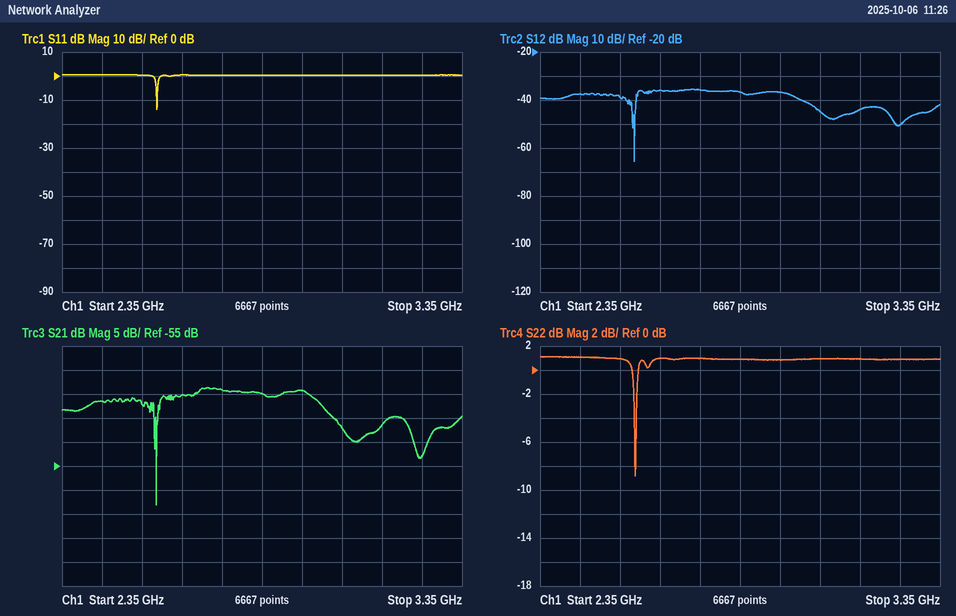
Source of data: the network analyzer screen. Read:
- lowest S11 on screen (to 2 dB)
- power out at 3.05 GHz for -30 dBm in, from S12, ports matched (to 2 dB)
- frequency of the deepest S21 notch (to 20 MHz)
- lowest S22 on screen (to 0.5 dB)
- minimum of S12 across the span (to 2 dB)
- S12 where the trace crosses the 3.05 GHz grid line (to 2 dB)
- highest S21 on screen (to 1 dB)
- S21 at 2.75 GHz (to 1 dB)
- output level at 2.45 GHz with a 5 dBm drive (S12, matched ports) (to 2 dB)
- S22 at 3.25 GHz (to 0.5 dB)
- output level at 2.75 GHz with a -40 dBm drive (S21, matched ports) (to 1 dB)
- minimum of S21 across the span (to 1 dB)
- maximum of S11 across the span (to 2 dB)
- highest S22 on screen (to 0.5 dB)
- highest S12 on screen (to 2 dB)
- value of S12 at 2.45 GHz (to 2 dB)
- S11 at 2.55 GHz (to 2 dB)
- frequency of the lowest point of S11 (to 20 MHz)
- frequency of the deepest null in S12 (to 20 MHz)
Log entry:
-14 dB
-74 dBm
2.58 GHz
-9.0 dB
-66 dB
-44 dB
-39 dB
-39 dB
-32 dBm
1.0 dB
-79 dBm
-63 dB
0 dB
1.0 dB
-36 dB
-38 dB
0 dB
2.58 GHz
2.58 GHz
